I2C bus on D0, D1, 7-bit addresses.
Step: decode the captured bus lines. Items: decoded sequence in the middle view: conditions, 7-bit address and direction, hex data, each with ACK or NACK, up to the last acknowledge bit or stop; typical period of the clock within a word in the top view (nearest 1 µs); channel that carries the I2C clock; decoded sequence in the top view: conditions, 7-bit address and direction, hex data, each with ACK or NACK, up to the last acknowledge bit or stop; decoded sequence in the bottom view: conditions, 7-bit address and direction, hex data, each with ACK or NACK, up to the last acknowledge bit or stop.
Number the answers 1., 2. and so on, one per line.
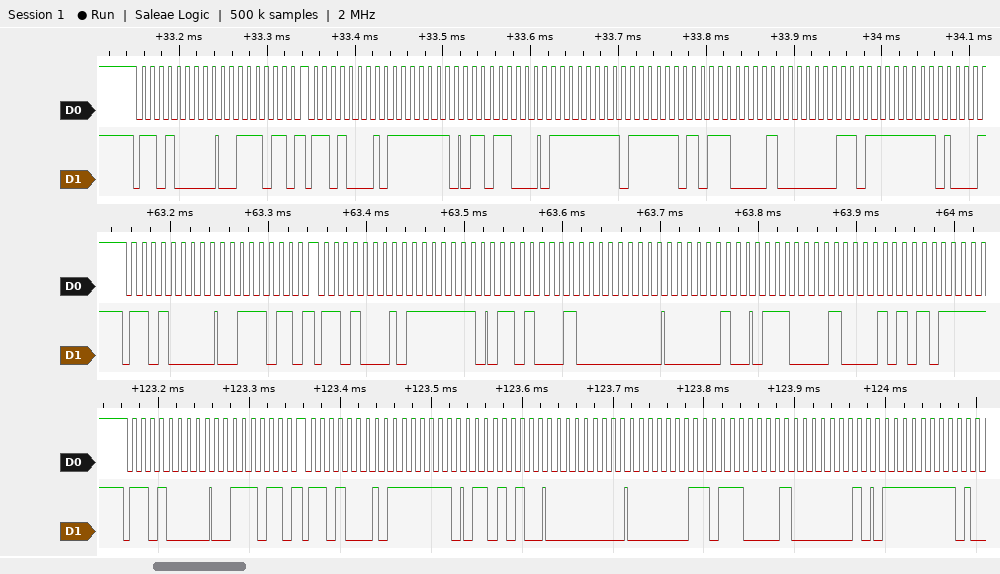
1. start, address 68 write ACK, 3B ACK, repeated start, address 68 read ACK, FE ACK, D1 ACK, 00 ACK, 04 ACK, E1 ACK, 15 ACK
2. 10 µs
3. D0
4. start, address 68 write ACK, 3B ACK, repeated start, address 68 read ACK, FE ACK, D8 ACK, FF ACK, FD ACK, E1 ACK, 03 ACK, FF ACK
5. start, address 68 write ACK, 3B ACK, repeated start, address 68 read ACK, FE ACK, D4 ACK, 00 ACK, 03 ACK, E1 ACK, 02 ACK, FF ACK
